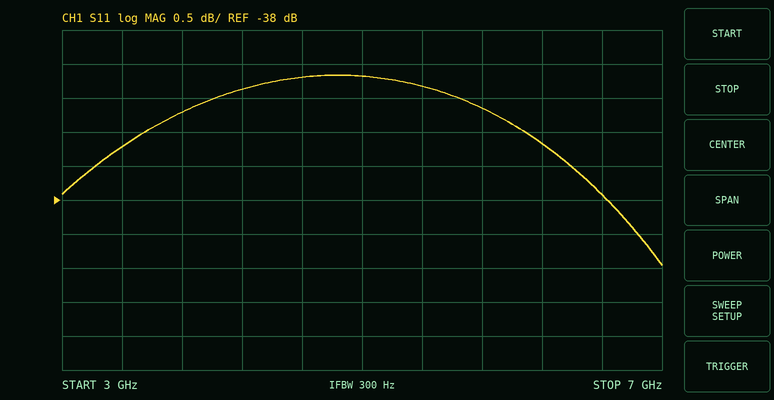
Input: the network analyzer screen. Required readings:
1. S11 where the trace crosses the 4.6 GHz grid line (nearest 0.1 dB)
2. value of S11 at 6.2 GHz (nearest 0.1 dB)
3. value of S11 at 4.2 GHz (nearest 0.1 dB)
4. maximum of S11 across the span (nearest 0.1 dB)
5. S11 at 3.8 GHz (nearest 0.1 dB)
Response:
-36.2 dB
-37.2 dB
-36.4 dB
-36.2 dB
-36.7 dB
